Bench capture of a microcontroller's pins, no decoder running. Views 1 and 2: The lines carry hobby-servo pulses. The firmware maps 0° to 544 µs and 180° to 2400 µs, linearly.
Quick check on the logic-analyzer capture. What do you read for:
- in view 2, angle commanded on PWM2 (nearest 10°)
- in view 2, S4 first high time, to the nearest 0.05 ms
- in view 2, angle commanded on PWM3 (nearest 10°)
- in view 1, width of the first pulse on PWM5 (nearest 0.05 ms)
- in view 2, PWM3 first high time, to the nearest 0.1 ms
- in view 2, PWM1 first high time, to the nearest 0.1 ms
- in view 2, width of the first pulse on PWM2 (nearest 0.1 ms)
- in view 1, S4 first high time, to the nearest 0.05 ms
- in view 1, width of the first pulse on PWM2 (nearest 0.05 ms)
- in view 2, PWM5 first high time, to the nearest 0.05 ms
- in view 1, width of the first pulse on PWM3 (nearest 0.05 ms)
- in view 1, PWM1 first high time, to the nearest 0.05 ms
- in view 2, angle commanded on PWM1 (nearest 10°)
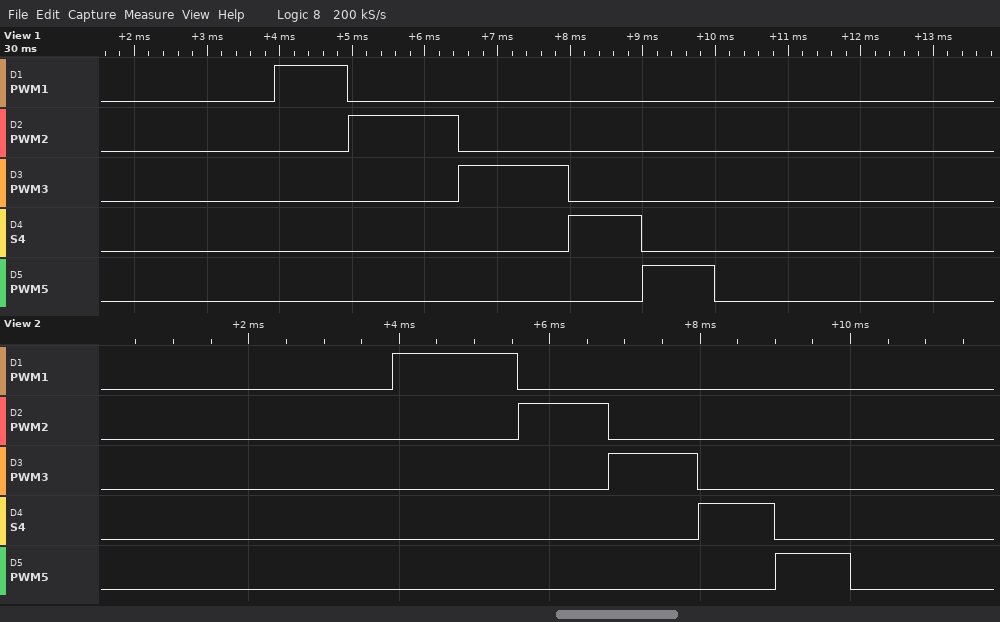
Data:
60°
1.00 ms
60°
1.00 ms
1.2 ms
1.7 ms
1.2 ms
1.00 ms
1.50 ms
1.00 ms
1.50 ms
1.00 ms
110°
